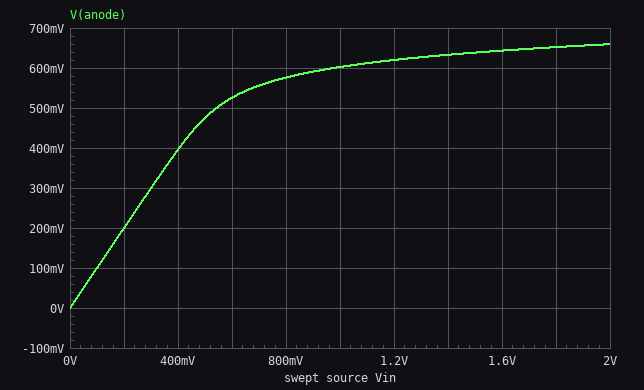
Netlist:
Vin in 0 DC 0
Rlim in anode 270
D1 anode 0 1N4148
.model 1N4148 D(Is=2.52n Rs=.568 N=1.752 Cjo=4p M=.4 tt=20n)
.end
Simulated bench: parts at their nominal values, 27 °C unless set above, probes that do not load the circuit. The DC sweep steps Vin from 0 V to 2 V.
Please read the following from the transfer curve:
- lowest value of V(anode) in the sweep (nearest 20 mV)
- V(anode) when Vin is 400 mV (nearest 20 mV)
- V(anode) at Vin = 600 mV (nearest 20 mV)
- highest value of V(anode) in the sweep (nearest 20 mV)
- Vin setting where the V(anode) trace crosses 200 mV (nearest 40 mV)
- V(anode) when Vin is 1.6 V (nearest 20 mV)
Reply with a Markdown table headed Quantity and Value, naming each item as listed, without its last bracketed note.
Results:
| Quantity | Value |
|---|---|
| lowest value of V(anode) in the sweep | 0 V |
| V(anode) when Vin is 400 mV | 400 mV |
| V(anode) at Vin = 600 mV | 520 mV |
| highest value of V(anode) in the sweep | 660 mV |
| Vin setting where the V(anode) trace crosses 200 mV | 200 mV |
| V(anode) when Vin is 1.6 V | 640 mV |
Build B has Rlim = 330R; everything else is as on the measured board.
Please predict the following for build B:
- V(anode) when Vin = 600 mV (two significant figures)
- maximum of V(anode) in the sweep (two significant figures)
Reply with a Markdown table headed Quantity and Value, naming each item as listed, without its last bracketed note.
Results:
| Quantity | Value |
|---|---|
| V(anode) when Vin = 600 mV | 520 mV |
| maximum of V(anode) in the sweep | 650 mV |
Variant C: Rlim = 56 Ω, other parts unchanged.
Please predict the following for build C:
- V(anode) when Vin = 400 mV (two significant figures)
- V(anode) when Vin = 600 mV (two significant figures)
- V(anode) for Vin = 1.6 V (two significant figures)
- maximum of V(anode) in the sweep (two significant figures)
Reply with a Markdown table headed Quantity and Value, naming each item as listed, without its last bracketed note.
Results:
| Quantity | Value |
|---|---|
| V(anode) when Vin = 400 mV | 400 mV |
| V(anode) when Vin = 600 mV | 560 mV |
| V(anode) for Vin = 1.6 V | 720 mV |
| maximum of V(anode) in the sweep | 740 mV |
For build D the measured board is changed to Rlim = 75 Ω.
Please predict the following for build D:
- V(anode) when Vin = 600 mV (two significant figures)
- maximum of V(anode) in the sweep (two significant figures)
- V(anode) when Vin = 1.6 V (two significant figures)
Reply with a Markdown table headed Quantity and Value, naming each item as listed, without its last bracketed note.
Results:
| Quantity | Value |
|---|---|
| V(anode) when Vin = 600 mV | 560 mV |
| maximum of V(anode) in the sweep | 720 mV |
| V(anode) when Vin = 1.6 V | 700 mV |
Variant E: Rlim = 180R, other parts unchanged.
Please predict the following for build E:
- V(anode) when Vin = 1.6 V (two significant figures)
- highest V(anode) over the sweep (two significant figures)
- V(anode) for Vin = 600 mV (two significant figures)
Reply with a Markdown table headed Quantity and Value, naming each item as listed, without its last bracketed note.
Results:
| Quantity | Value |
|---|---|
| V(anode) when Vin = 1.6 V | 660 mV |
| highest V(anode) over the sweep | 680 mV |
| V(anode) for Vin = 600 mV | 540 mV |
